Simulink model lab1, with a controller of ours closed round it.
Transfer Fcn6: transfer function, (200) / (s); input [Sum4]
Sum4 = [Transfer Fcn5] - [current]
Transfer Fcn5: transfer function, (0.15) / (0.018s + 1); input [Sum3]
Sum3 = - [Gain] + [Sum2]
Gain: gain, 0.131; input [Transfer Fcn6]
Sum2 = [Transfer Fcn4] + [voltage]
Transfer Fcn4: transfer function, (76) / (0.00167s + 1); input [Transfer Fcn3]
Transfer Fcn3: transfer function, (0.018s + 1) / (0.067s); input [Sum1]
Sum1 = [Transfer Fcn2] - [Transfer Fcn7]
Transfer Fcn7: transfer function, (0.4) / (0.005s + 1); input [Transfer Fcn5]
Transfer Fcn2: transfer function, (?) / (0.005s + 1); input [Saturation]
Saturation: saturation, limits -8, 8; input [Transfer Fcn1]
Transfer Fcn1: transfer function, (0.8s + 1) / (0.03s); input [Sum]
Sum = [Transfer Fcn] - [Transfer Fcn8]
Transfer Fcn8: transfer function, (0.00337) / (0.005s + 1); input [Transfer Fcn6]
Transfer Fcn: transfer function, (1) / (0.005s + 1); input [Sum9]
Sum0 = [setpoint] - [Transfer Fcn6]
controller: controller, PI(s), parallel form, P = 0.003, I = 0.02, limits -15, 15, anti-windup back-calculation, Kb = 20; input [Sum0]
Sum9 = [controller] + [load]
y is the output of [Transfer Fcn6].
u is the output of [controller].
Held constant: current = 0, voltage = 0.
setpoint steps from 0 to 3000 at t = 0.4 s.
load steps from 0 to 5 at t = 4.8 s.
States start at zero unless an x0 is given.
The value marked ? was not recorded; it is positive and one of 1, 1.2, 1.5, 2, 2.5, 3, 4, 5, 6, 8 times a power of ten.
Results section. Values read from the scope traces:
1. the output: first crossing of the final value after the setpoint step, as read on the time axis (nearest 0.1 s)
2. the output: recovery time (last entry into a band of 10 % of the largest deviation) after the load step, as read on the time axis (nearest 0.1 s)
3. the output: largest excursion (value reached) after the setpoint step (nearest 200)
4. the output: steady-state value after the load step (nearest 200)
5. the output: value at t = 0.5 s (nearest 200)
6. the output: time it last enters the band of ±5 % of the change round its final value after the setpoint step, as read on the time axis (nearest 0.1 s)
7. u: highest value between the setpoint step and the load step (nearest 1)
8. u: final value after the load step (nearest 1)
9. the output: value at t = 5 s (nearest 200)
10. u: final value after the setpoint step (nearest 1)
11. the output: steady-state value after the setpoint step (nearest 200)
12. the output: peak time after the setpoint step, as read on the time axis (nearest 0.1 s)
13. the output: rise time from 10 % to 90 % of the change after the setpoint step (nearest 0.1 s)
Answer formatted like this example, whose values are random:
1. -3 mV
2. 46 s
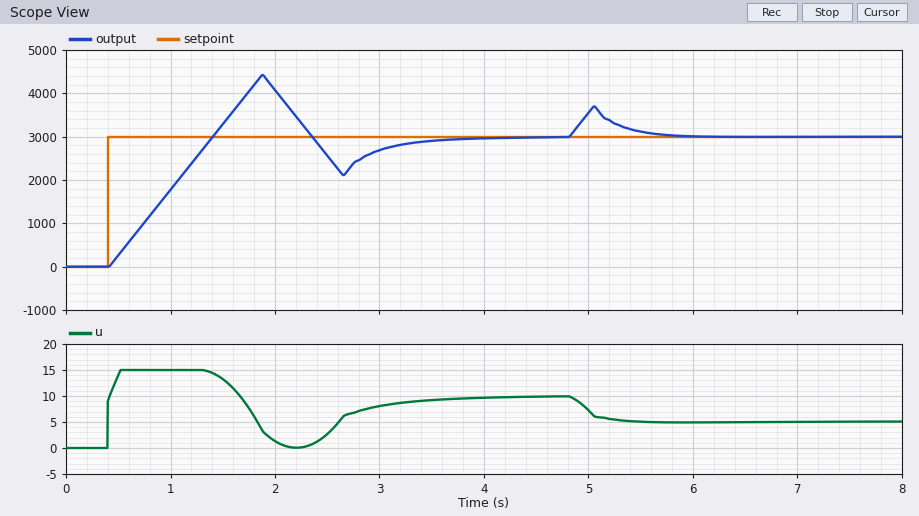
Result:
1. 1.4 s
2. 5.6 s
3. 4400
4. 3000
5. 200
6. 3.3 s
7. 15
8. 5
9. 3600
10. 10
11. 3000
12. 1.9 s
13. 0.8 s
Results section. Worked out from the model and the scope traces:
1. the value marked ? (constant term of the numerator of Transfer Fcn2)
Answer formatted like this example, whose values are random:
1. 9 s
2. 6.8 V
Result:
1. 0.8
